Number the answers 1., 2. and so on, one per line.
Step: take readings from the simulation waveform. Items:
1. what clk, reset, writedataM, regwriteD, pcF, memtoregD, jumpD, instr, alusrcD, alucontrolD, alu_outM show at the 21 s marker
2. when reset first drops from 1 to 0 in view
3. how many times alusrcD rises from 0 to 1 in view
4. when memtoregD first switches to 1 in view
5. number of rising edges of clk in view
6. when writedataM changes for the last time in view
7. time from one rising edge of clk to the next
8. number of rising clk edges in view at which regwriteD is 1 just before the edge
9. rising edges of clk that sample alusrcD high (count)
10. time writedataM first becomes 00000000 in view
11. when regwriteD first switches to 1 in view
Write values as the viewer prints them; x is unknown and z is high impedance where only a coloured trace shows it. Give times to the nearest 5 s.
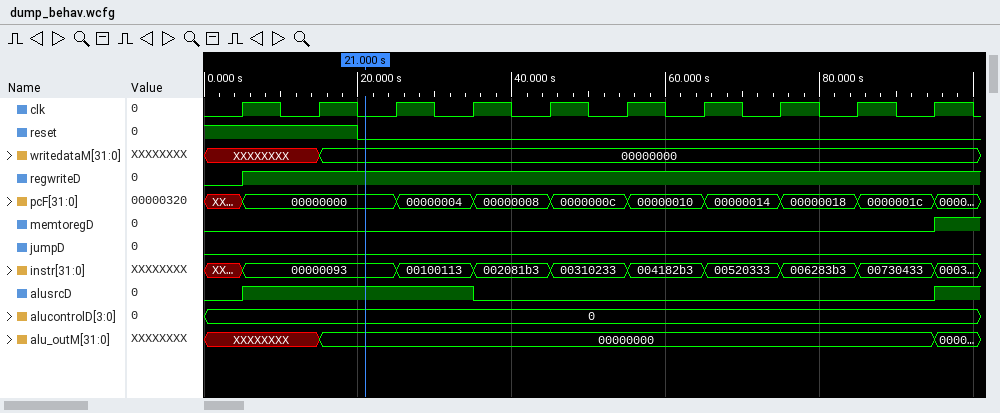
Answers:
1. clk=0, reset=0, writedataM=00000000, regwriteD=1, pcF=00000000, memtoregD=0, jumpD=0, instr=00000093, alusrcD=1, alucontrolD=0, alu_outM=00000000
2. 20 s
3. 2
4. 95 s
5. 10
6. 15 s
7. 10 s
8. 9
9. 3
10. 15 s
11. 5 s
